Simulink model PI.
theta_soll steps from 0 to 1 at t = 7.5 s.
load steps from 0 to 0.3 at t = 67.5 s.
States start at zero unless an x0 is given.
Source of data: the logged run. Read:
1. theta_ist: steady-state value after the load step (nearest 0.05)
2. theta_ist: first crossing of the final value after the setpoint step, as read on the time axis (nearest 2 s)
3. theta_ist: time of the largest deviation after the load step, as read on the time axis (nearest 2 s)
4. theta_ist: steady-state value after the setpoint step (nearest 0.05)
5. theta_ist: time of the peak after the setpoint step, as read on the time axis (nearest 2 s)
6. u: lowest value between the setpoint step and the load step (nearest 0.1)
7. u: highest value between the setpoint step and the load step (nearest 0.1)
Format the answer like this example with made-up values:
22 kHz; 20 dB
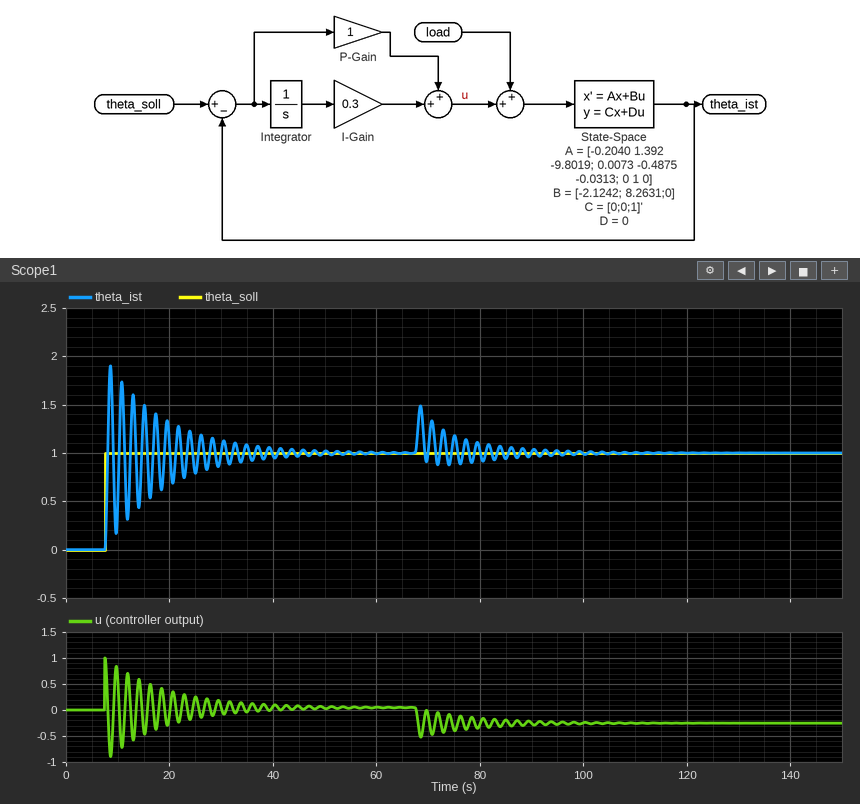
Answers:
1.00; 8 s; 68 s; 1.00; 8 s; -0.9; 1.0
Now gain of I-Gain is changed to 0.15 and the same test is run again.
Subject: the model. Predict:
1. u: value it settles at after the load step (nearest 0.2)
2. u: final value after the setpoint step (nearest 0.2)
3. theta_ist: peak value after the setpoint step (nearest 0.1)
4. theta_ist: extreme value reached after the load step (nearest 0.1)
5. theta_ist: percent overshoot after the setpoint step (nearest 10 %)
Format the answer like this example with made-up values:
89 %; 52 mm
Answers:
-0.2; 0.0; 1.8; 1.5; 80 %
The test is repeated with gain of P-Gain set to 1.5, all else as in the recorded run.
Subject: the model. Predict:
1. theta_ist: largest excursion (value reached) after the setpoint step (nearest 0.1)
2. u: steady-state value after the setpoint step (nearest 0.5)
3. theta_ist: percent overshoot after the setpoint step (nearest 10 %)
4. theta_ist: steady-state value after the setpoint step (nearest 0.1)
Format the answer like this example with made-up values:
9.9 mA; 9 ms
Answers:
1.9; 0.0; 90 %; 1.0
